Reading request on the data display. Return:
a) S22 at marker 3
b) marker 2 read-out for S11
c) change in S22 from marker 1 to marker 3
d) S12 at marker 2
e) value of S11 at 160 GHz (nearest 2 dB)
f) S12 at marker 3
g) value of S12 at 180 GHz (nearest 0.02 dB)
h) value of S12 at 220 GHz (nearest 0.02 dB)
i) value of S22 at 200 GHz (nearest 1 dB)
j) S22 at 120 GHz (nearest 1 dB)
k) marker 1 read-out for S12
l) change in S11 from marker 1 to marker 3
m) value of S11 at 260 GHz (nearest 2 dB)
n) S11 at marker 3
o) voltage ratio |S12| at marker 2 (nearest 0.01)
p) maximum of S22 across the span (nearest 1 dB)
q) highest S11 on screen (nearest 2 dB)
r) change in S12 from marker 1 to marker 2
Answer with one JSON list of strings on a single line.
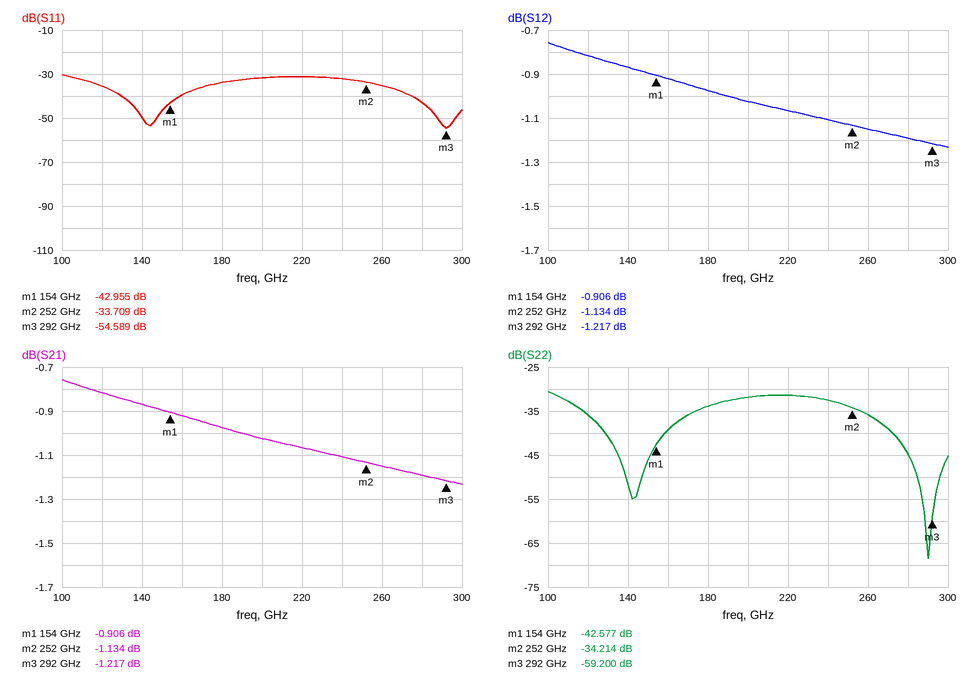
["-59.200 dB", "-33.709 dB", "-16.623 dB", "-1.134 dB", "-40 dB", "-1.217 dB", "-0.98 dB", "-1.06 dB", "-32 dB", "-36 dB", "-0.906 dB", "-11.634 dB", "-36 dB", "-54.589 dB", "0.88", "-31 dB", "-30 dB", "-0.228 dB"]
